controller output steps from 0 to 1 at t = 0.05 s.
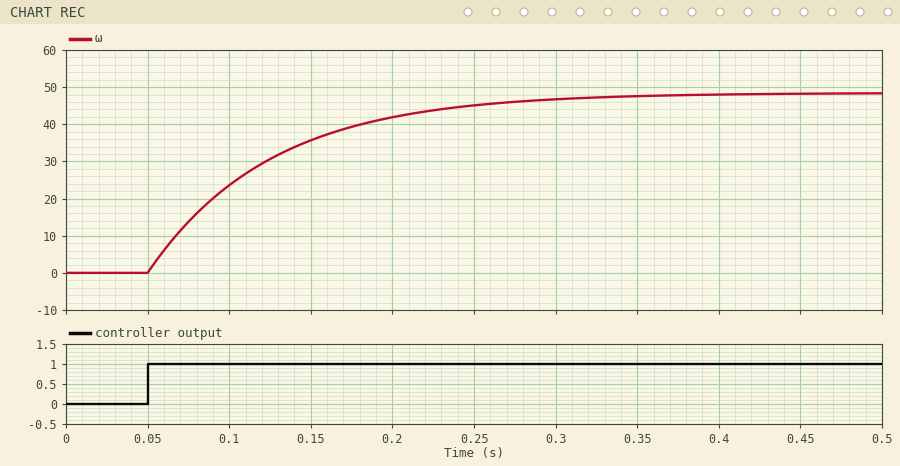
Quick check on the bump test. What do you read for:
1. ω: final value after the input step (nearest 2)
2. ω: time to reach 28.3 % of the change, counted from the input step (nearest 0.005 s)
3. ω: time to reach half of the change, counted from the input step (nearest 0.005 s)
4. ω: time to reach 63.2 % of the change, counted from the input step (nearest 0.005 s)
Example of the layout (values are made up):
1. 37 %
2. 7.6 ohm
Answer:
1. 48
2. 0.025 s
3. 0.050 s
4. 0.075 s
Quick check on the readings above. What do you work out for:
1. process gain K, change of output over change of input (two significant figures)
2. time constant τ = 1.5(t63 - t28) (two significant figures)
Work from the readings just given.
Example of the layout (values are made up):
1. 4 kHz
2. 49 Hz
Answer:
1. 48
2. 0.075 s
